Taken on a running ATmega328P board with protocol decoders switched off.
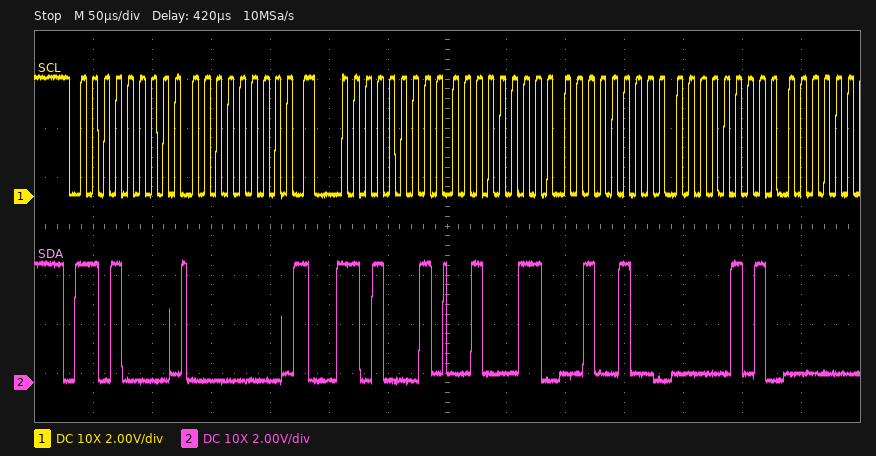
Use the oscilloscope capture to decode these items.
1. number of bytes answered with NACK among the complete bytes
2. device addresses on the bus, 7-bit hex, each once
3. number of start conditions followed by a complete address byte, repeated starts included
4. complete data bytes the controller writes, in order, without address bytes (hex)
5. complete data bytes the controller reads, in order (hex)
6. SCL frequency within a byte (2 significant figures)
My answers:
0
0x68
2
00
23 24 05
100 kHz
